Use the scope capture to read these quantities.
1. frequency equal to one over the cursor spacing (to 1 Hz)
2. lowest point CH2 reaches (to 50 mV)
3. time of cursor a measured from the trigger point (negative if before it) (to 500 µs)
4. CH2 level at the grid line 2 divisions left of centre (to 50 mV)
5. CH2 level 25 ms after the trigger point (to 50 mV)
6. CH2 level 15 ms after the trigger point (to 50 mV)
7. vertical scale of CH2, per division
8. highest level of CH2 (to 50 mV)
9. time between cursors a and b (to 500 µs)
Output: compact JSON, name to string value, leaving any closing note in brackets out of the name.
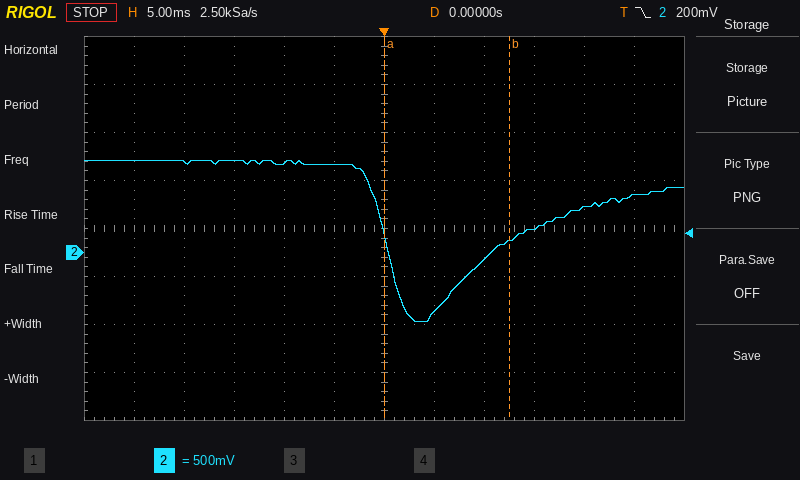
{"frequency equal to one over the cursor spacing": "80 Hz", "lowest point CH2 reaches": "-700 mV", "time of cursor a measured from the trigger point (negative if before it)": "0.0 ms", "CH2 level at the grid line 2 divisions left of centre": "950 mV", "CH2 level 25 ms after the trigger point": "600 mV", "CH2 level 15 ms after the trigger point": "250 mV", "vertical scale of CH2, per division": "500 mV", "highest level of CH2": "950 mV", "time between cursors a and b": "12.5 ms"}
